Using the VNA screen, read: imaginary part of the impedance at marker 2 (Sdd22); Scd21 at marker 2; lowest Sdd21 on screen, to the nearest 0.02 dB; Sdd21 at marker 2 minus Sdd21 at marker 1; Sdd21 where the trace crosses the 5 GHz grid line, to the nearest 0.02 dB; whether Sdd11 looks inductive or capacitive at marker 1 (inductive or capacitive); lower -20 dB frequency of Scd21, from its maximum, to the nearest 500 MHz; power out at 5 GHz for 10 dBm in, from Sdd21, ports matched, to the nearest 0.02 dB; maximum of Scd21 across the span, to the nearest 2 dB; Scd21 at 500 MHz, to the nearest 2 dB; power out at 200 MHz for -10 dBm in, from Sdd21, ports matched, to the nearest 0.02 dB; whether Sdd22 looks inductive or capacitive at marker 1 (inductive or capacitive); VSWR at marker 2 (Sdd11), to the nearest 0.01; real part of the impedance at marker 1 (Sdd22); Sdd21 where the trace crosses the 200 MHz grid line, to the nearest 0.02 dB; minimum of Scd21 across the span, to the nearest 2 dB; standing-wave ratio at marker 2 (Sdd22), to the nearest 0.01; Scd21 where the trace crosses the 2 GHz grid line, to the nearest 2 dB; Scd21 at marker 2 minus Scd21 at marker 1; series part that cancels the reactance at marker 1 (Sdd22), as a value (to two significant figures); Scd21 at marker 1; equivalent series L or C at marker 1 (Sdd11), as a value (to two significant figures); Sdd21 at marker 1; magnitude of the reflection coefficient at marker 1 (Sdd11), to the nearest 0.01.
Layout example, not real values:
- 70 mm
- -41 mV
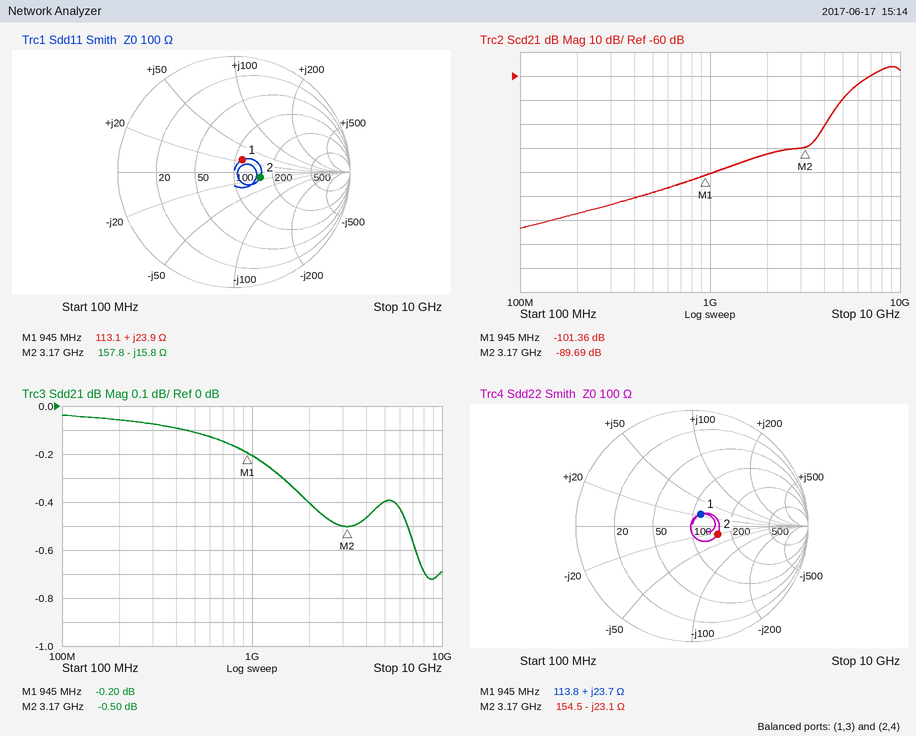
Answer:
- -23.1 Ω
- -89.69 dB
- -0.72 dB
- -0.30 dB
- -0.40 dB
- inductive
- 4.5 GHz
- 9.60 dBm
- -56 dB
- -108 dB
- -10.06 dBm
- inductive
- 1.60
- 113.8 Ω
- -0.06 dB
- -124 dB
- 1.60
- -92 dB
- 11.67 dB
- 7.1 pF
- -101.36 dB
- 4.0 nH
- -0.20 dB
- 0.13
